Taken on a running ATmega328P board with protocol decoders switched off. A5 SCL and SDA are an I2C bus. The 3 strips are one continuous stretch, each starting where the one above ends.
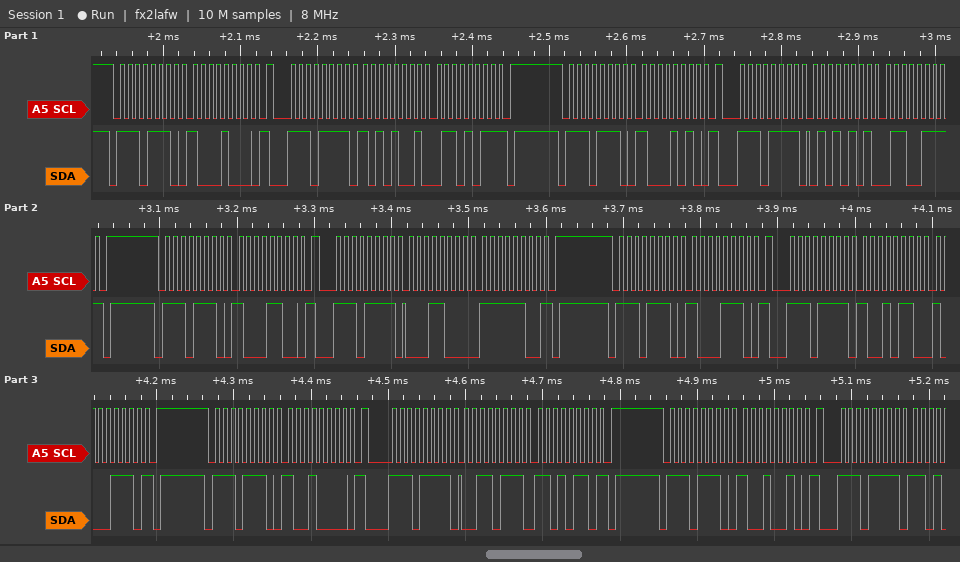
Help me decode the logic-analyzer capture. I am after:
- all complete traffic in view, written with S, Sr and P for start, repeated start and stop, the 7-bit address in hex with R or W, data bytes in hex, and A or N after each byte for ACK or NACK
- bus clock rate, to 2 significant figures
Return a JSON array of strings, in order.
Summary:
["S 77W A 88 A Sr 77R A A9 A 6B N P S 77W A 8A A Sr 77R A 55 A 67 N P S 77W A 8C A Sr 77R A 18 A FC N P S 77W A 8E A Sr 77R A 96 A 8E N P S 77W A 90 A Sr 77R A 37 A D6 N P S 77W A 92 A Sr 77R A", "100 kHz"]
